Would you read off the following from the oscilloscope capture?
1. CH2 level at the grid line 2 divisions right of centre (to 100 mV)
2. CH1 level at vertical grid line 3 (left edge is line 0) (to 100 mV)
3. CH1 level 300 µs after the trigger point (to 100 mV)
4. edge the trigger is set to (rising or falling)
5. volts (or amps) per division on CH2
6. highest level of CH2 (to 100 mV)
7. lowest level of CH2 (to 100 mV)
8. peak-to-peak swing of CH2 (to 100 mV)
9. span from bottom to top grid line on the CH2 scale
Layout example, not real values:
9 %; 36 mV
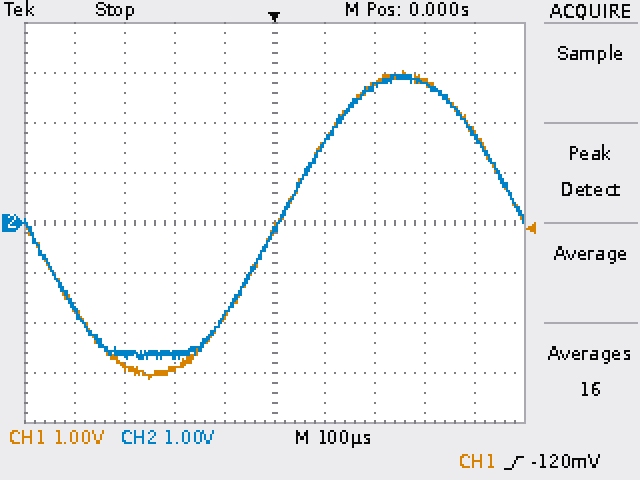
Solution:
2.7 V; -2.9 V; 2.8 V; rising; 1 V; 3.0 V; -2.7 V; 5.7 V; 8 V
